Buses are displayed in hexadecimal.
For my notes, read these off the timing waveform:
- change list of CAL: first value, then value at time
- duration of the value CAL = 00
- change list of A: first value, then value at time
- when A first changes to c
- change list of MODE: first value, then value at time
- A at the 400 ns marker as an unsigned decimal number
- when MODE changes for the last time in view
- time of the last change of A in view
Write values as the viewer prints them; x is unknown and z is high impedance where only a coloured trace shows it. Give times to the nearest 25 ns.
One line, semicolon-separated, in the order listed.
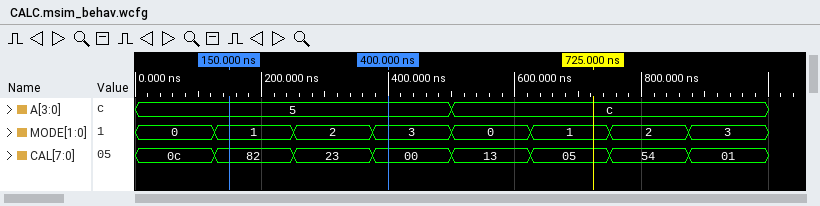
0c, 82 at 125 ns, 23 at 250 ns, 00 at 375 ns, 13 at 500 ns, 05 at 625 ns, 54 at 750 ns, 01 at 875 ns; 125 ns; 5, c at 500 ns; 500 ns; 0, 1 at 125 ns, 2 at 250 ns, 3 at 375 ns, 0 at 500 ns, 1 at 625 ns, 2 at 750 ns, 3 at 875 ns; 5; 875 ns; 500 ns
